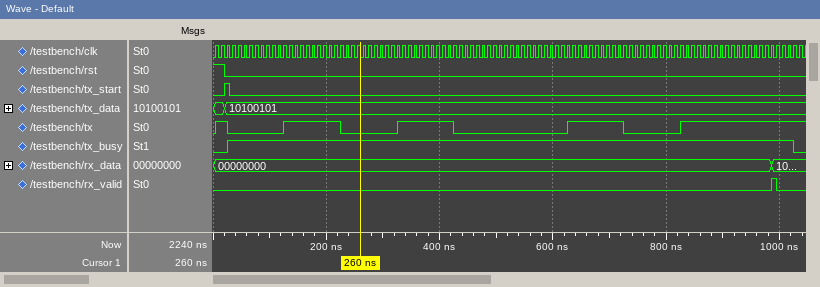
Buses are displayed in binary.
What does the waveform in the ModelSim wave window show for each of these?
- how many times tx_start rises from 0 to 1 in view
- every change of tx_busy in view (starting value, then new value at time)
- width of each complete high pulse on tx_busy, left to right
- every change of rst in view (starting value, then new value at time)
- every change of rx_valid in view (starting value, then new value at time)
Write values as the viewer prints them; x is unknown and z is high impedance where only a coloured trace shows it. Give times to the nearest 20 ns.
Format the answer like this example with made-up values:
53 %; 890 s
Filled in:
1; 0, 1 at 20 ns, 0 at 1020 ns; 1000 ns; 1, 0 at 20 ns; 0, 1 at 980 ns, 0 at 1000 ns
